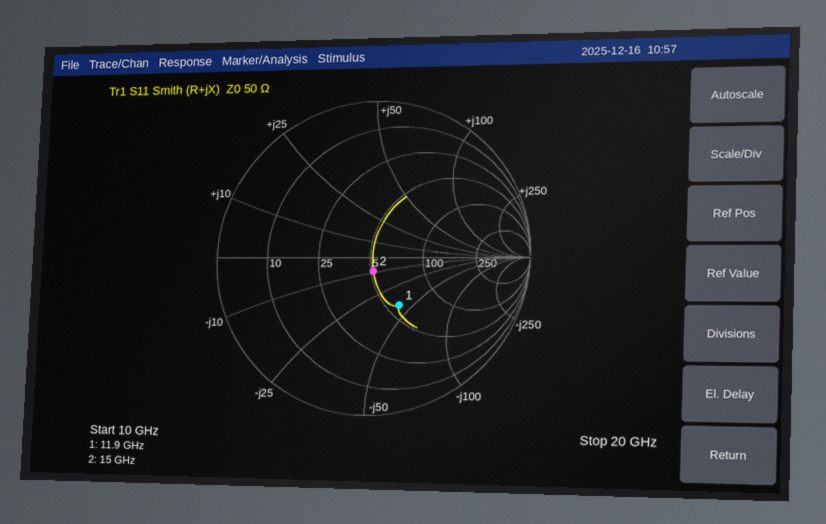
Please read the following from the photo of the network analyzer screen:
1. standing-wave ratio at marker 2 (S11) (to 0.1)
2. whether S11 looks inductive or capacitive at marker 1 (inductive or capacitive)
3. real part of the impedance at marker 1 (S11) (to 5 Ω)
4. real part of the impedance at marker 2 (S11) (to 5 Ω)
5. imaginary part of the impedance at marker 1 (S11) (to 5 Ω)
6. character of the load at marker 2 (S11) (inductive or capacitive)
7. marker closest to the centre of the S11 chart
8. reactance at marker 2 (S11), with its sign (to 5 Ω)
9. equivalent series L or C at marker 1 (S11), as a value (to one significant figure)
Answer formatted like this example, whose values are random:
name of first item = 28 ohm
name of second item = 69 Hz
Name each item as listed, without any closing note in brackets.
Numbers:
standing-wave ratio at marker 2 (S11) = 1.2
whether S11 looks inductive or capacitive at marker 1 = capacitive
real part of the impedance at marker 1 (S11) = 60 Ω
real part of the impedance at marker 2 (S11) = 50 Ω
imaginary part of the impedance at marker 1 (S11) = -40 Ω
character of the load at marker 2 (S11) = capacitive
marker closest to the centre of the S11 chart = marker 2
reactance at marker 2 (S11), with its sign = -10 Ω
equivalent series L or C at marker 1 (S11), as a value = 300 fF
